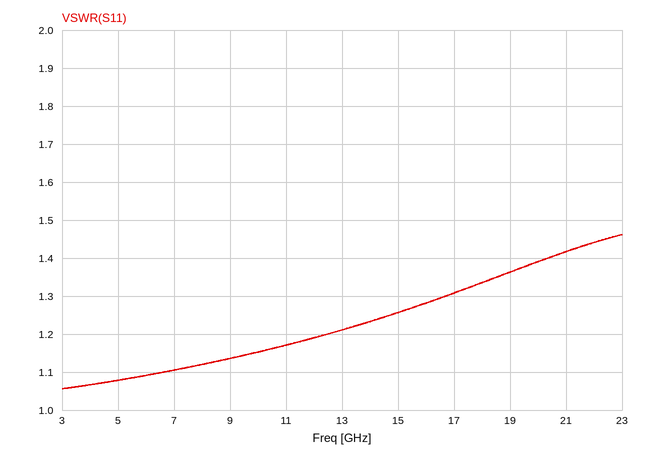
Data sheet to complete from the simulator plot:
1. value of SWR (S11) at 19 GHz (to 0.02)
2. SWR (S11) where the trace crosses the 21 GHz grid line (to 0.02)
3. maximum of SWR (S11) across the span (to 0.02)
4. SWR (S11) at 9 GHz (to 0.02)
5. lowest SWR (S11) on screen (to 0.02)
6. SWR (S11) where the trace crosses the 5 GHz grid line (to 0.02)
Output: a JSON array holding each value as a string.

["1.36", "1.42", "1.46", "1.14", "1.06", "1.08"]
